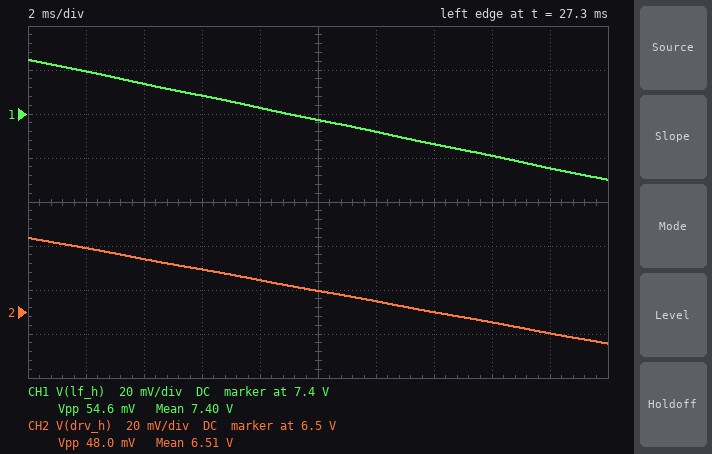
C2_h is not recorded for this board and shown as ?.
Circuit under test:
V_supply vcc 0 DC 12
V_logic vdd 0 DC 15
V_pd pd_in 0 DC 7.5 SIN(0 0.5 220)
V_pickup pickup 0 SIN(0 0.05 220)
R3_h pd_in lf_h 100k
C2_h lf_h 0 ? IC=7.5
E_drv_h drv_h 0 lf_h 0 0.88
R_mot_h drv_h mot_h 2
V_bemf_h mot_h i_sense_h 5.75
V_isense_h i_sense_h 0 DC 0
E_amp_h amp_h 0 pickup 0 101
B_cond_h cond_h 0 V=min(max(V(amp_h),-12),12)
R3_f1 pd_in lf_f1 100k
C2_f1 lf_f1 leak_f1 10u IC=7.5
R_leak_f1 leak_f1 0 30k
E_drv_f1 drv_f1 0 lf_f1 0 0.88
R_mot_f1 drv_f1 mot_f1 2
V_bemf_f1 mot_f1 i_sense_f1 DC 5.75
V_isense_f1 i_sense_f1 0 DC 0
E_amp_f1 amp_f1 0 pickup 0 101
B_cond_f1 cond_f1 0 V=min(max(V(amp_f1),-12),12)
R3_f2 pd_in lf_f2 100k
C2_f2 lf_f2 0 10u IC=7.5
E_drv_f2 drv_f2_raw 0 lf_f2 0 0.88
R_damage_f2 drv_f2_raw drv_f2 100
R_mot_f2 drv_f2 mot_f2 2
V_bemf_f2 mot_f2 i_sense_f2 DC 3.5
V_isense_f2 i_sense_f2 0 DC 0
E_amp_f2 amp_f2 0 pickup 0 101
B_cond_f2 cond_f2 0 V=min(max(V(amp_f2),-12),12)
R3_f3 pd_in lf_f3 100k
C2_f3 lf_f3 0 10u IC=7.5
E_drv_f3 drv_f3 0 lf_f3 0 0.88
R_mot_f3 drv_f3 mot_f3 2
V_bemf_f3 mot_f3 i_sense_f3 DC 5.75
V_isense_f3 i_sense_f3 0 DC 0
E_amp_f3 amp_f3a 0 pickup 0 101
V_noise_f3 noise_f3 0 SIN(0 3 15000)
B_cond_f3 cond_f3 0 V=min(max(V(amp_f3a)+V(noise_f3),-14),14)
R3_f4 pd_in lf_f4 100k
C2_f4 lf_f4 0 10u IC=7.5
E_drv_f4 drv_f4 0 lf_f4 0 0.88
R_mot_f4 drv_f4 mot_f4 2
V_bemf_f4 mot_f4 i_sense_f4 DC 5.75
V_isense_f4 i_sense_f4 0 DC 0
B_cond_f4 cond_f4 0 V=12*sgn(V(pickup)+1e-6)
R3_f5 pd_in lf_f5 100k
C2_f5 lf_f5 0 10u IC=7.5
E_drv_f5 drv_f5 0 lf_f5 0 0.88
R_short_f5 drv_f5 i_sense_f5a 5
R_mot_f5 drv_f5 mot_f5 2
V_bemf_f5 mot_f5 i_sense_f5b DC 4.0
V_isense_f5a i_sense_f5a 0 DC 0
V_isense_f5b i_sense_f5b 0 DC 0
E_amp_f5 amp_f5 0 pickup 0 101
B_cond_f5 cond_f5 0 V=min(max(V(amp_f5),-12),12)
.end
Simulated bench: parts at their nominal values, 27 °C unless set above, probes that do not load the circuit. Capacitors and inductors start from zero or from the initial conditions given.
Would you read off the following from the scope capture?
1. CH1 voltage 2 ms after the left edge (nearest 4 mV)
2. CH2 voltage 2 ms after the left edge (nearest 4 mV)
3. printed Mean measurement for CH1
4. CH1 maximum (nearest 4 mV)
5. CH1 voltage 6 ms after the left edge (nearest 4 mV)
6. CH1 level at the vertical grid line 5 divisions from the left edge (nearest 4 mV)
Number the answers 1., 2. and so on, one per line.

1. 7.420 V
2. 6.528 V
3. 7.40 V
4. 7.424 V
5. 7.408 V
6. 7.396 V
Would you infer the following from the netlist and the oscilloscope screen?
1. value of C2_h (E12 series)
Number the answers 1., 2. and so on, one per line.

1. 27 µF
